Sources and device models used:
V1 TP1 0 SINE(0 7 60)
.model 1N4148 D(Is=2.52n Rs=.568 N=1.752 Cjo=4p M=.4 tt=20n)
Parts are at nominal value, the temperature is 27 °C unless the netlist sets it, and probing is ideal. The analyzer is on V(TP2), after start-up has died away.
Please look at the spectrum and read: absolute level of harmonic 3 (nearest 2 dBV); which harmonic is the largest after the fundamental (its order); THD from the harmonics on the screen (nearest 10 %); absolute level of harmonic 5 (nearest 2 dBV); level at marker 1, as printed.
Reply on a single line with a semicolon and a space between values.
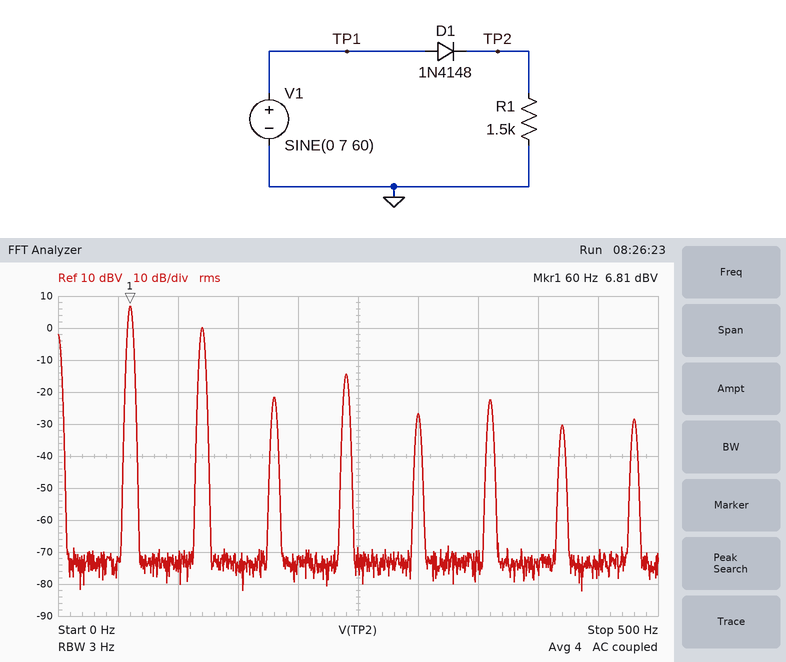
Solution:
-22 dBV; 2; 50 %; -26 dBV; 6.81 dBV
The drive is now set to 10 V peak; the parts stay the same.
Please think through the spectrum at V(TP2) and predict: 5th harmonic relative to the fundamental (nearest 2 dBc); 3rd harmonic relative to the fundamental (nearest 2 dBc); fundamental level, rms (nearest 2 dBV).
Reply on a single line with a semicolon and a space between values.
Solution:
-36 dBc; -32 dBc; 10 dBV
